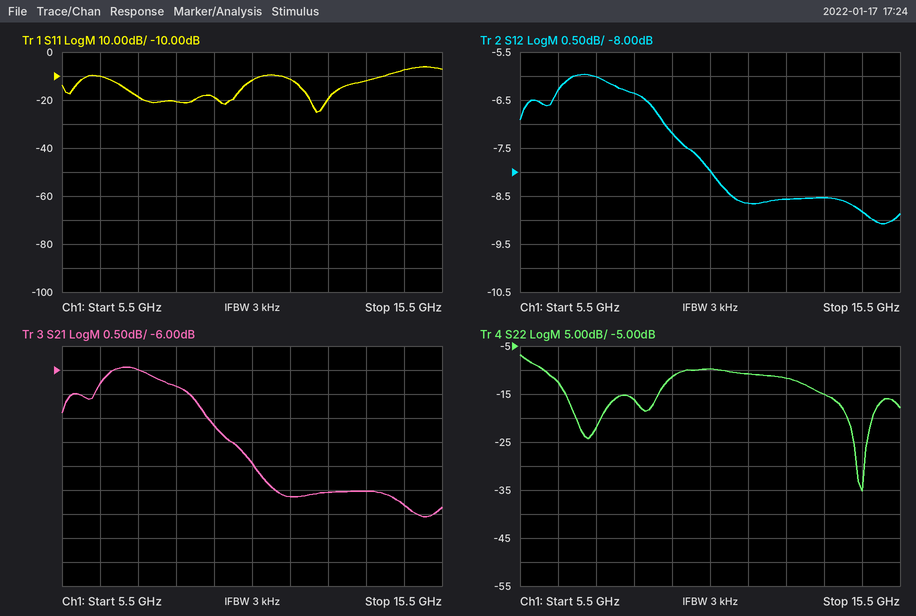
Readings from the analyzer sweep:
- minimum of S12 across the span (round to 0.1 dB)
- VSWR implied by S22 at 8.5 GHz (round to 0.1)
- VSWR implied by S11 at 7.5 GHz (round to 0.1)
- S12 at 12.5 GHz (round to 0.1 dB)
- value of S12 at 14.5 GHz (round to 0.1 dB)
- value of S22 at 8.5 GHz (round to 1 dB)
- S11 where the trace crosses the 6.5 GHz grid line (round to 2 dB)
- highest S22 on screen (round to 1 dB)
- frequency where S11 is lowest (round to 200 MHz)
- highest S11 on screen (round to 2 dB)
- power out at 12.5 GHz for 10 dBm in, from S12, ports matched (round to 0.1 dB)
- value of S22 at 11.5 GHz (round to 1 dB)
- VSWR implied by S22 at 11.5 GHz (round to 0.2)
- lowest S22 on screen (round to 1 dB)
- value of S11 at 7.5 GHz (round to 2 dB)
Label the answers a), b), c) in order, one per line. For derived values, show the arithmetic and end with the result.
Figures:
a) -9.1 dB
b) |Γ| = 10^(-16/20) = 0.1585; VSWR = (1 + 0.1585)/(1 − 0.1585) ≈ 1.4
c) |Γ| = 10^(-18/20) = 0.1259; VSWR = (1 + 0.1259)/(1 − 0.1259) ≈ 1.3
d) -8.6 dB
e) -8.8 dB
f) -16 dB
g) -10 dB
h) -7 dB
i) 12.2 GHz
j) -6 dB
k) 10 dBm + (-8.6 dB) = 1.4 dBm
l) -11 dB
m) |Γ| = 10^(-11/20) = 0.2818; VSWR = (1 + 0.2818)/(1 − 0.2818) ≈ 1.8
n) -35 dB
o) -18 dB
